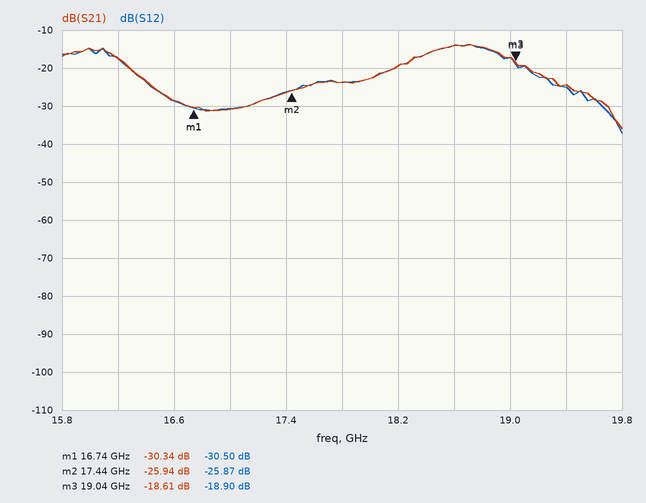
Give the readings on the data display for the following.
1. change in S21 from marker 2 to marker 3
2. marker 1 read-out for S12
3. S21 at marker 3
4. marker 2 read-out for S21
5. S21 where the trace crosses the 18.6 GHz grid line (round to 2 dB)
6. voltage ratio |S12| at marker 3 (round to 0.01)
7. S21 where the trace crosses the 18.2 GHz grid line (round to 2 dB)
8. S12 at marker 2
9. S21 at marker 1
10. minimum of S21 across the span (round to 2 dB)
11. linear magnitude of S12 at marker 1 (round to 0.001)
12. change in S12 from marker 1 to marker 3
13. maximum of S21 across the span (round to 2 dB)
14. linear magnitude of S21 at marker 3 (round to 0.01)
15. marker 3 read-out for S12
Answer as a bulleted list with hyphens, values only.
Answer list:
- 7.33 dB
- -30.50 dB
- -18.61 dB
- -25.94 dB
- -14 dB
- 0.11
- -20 dB
- -25.87 dB
- -30.34 dB
- -36 dB
- 0.030
- 11.60 dB
- -14 dB
- 0.12
- -18.90 dB
